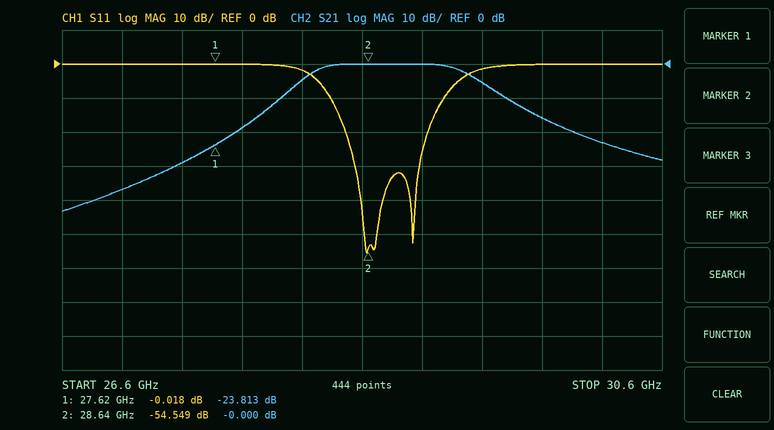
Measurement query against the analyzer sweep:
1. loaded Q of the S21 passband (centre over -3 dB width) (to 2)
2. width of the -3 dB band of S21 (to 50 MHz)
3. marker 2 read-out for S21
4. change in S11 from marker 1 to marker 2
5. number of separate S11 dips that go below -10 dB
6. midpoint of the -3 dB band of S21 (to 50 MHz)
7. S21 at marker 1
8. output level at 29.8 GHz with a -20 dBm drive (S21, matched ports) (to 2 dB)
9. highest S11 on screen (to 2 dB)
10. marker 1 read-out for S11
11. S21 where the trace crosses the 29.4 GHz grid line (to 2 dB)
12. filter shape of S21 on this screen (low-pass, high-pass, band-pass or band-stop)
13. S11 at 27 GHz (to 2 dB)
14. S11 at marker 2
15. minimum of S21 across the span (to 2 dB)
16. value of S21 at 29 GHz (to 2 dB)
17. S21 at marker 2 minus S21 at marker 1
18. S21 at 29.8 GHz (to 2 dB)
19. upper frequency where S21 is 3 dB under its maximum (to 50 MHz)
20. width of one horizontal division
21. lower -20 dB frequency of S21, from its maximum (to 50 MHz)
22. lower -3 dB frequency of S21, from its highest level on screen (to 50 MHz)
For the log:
28
1.05 GHz
-0.000 dB
-54.531 dB
2
28.80 GHz
-23.813 dB
-36 dBm
0 dB
-0.018 dB
-6 dB
band-pass
0 dB
-54.549 dB
-44 dB
0 dB
23.813 dB
-16 dB
29.30 GHz
400 MHz
27.75 GHz
28.25 GHz
